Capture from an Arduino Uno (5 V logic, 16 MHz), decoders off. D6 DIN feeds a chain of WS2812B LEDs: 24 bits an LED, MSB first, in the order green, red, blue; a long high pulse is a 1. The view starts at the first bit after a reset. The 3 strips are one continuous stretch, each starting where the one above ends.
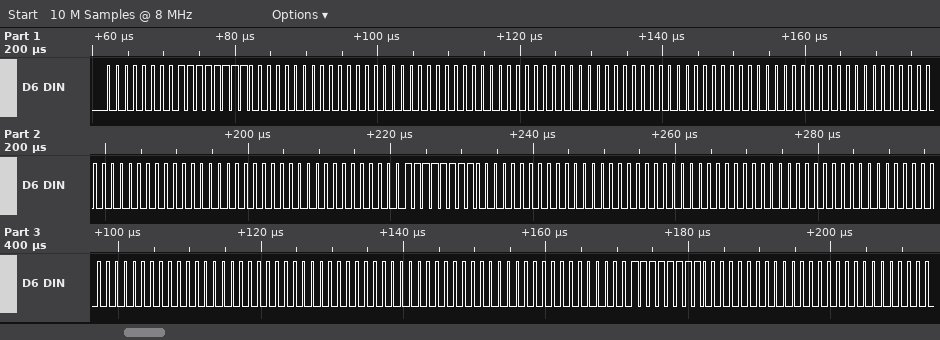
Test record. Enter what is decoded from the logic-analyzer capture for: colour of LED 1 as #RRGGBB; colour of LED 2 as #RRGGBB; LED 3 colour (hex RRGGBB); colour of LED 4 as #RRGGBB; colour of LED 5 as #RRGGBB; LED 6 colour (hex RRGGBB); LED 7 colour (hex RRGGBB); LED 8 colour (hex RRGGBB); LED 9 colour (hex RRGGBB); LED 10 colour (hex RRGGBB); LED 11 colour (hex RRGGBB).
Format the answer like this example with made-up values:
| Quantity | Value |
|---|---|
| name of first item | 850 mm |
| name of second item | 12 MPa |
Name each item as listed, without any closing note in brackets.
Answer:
| Quantity | Value |
|---|---|
| colour of LED 1 as #RRGGBB | #FF0000 |
| colour of LED 2 as #RRGGBB | #000000 |
| LED 3 colour | #000000 |
| colour of LED 4 as #RRGGBB | #000000 |
| colour of LED 5 as #RRGGBB | #000000 |
| LED 6 colour | #FF0000 |
| LED 7 colour | #000000 |
| LED 8 colour | #000000 |
| LED 9 colour | #000000 |
| LED 10 colour | #000000 |
| LED 11 colour | #FF0000 |
